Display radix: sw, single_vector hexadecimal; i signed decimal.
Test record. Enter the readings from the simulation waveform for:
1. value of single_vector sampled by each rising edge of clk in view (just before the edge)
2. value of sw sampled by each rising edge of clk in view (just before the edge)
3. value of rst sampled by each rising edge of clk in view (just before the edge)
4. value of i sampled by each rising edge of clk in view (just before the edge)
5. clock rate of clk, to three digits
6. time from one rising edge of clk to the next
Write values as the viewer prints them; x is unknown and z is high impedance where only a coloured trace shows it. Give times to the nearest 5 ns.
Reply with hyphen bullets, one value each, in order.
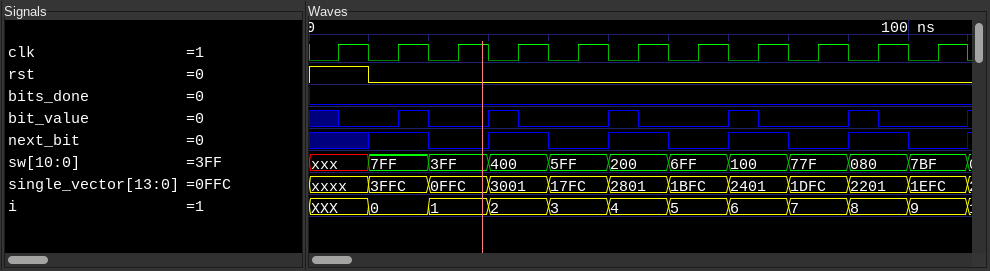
- xxxx, 3FFC, 0FFC, 3001, 17FC, 2801, 1BFC, 2401, 1DFC, 2201, 1EFC
- xxx, 7FF, 3FF, 400, 5FF, 200, 6FF, 100, 77F, 080, 7BF
- 1 0 0 0 0 0 0 0 0 0 0
- XXX, 0, 1, 2, 3, 4, 5, 6, 7, 8, 9
- 100 MHz
- 10 ns
